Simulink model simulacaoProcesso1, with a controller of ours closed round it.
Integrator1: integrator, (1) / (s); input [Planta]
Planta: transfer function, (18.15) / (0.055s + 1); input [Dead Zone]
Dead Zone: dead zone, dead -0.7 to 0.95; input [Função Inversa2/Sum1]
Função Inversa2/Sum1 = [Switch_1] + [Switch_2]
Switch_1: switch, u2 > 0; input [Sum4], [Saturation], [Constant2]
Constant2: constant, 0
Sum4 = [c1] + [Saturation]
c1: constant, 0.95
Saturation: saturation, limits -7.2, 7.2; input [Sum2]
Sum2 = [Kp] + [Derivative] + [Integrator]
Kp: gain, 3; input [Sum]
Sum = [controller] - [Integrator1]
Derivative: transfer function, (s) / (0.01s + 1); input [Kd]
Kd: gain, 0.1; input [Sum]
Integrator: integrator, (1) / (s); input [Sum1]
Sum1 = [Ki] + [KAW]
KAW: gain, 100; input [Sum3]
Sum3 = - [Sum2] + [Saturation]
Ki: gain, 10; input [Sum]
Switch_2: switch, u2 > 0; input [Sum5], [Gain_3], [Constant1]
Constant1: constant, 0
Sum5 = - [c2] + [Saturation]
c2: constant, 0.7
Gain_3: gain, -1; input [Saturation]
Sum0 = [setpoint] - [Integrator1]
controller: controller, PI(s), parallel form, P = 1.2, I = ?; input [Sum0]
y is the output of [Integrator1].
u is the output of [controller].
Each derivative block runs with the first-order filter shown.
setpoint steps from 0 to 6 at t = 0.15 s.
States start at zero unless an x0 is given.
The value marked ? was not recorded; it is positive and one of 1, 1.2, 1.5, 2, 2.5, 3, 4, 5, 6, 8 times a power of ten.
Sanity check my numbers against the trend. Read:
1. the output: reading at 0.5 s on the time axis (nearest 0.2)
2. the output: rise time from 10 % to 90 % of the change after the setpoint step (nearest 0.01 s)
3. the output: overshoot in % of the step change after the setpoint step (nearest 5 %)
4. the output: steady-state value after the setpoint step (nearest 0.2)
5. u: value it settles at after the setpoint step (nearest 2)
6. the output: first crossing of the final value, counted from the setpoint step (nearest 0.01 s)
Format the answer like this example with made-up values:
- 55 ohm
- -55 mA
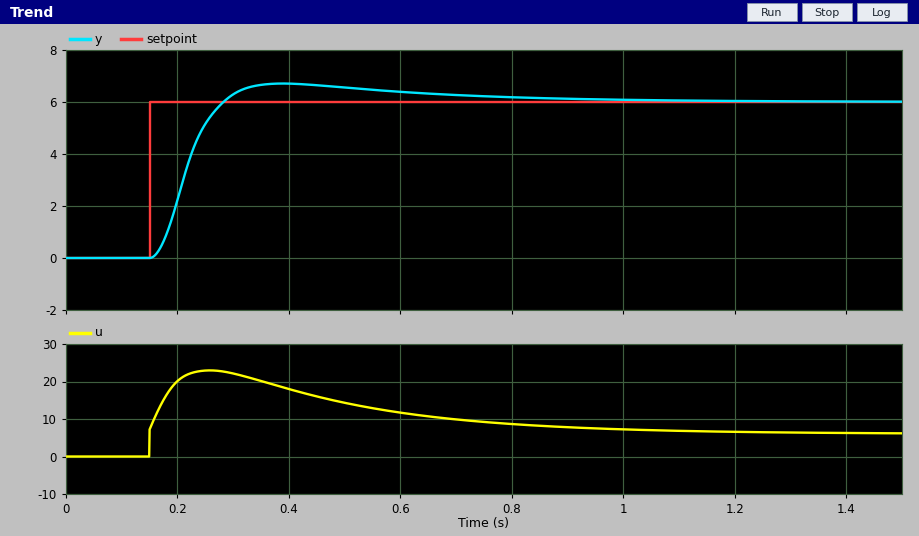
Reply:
- 6.6
- 0.08 s
- 10 %
- 6.0
- 6
- 0.13 s
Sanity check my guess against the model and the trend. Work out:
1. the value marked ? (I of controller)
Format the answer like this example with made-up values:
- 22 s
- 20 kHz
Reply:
- 60
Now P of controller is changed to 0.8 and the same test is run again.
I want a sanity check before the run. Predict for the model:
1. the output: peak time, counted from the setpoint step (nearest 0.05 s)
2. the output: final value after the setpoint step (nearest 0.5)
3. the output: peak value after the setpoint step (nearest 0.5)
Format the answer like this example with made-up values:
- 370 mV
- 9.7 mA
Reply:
- 0.20 s
- 6.0
- 6.5
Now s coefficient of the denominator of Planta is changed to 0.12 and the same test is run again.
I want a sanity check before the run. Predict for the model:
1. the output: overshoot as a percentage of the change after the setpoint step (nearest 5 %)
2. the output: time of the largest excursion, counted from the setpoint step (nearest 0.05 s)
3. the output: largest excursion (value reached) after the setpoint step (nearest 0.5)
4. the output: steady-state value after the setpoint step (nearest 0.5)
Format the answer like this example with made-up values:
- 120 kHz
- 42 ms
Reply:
- 15 %
- 0.30 s
- 7.0
- 6.0
